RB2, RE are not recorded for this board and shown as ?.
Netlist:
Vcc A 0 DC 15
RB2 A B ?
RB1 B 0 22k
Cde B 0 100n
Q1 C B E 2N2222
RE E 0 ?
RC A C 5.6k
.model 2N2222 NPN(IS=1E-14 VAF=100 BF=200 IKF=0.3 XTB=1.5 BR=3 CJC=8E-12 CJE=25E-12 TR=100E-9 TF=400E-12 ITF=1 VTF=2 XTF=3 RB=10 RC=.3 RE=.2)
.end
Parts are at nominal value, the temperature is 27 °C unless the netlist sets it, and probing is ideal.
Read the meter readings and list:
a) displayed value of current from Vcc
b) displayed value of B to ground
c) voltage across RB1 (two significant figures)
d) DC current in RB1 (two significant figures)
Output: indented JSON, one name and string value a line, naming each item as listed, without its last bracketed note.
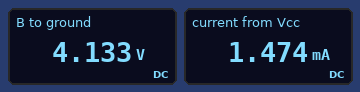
{
  "displayed value of current from Vcc": "1.474 mA",
  "displayed value of B to ground": "4.133 V",
  "voltage across RB1": "4.1 V",
  "DC current in RB1": "190 µA"
}
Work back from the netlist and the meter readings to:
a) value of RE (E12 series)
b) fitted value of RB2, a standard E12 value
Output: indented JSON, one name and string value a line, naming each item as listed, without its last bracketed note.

{
  "value of RE": "2.7 kΩ",
  "fitted value of RB2, a standard E12 value": "56 kΩ"
}
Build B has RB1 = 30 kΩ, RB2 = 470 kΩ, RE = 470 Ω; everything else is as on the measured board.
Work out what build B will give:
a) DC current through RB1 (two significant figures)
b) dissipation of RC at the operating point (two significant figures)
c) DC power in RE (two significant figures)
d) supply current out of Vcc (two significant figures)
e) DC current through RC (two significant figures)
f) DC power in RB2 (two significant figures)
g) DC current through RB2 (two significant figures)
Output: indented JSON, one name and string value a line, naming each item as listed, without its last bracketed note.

{
  "DC current through RB1": "28 µA",
  "dissipation of RC at the operating point": "1.1 mW",
  "DC power in RE": "95 µW",
  "supply current out of Vcc": "480 µA",
  "DC current through RC": "450 µA",
  "DC power in RB2": "430 µW",
  "DC current through RB2": "30 µA"
}
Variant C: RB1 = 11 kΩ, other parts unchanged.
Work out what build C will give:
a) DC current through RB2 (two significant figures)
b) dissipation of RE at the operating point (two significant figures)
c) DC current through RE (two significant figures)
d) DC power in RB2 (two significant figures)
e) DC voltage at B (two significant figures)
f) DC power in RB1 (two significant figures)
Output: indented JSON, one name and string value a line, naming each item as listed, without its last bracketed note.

{
  "DC current through RB2": "220 µA",
  "dissipation of RE at the operating point": "1.2 mW",
  "DC current through RE": "660 µA",
  "DC power in RB2": "2.8 mW",
  "DC voltage at B": "2.4 V",
  "DC power in RB1": "540 µW"
}
